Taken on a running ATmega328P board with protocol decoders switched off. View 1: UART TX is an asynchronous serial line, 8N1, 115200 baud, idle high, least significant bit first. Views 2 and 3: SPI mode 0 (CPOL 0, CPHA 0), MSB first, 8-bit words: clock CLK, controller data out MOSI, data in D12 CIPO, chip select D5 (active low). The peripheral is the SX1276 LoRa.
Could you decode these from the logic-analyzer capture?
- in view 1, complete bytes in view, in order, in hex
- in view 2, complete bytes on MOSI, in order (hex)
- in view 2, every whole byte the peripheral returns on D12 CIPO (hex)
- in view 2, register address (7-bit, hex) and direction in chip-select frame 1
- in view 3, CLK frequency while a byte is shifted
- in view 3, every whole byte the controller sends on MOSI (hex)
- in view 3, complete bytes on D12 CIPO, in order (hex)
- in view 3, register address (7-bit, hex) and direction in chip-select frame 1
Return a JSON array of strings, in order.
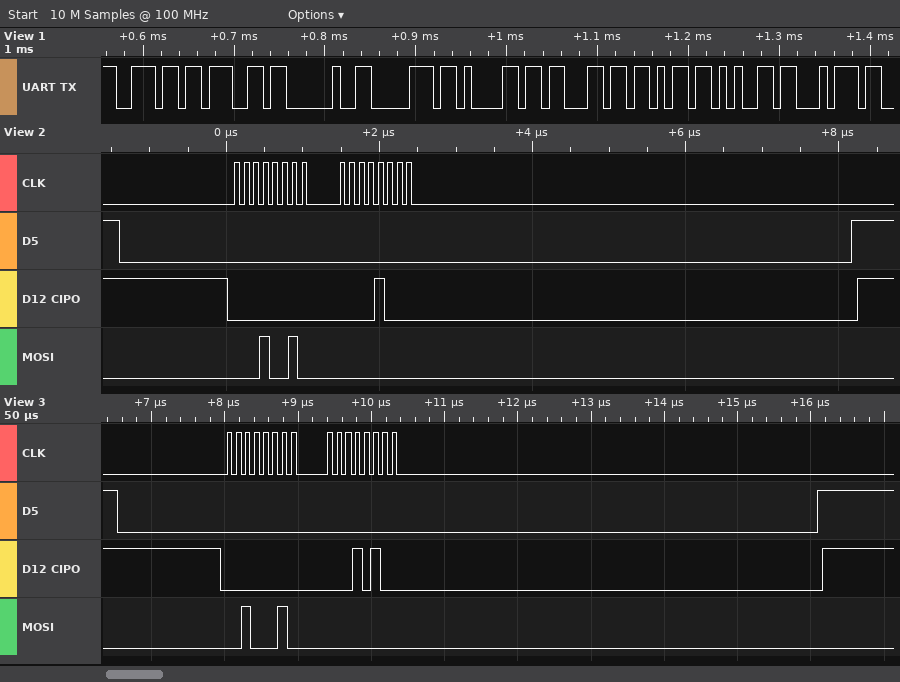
["6E 67 20 70 61 63 6B 65 74", "12 00", "00 08", "0x12 read", "8 MHz", "0x22 0x00", "0x00 0x14", "0x22 read"]
